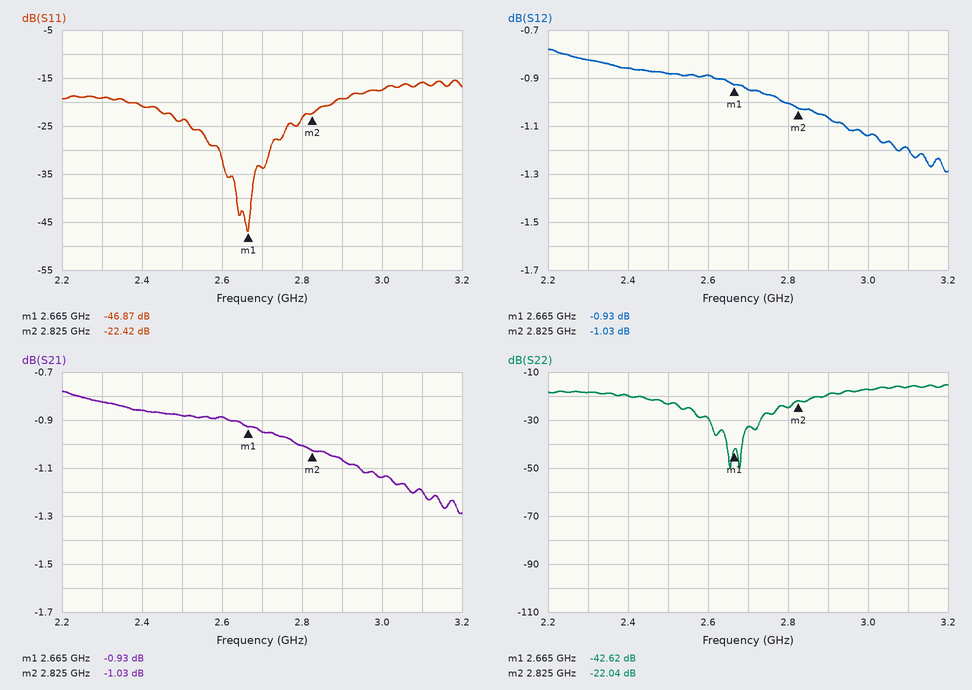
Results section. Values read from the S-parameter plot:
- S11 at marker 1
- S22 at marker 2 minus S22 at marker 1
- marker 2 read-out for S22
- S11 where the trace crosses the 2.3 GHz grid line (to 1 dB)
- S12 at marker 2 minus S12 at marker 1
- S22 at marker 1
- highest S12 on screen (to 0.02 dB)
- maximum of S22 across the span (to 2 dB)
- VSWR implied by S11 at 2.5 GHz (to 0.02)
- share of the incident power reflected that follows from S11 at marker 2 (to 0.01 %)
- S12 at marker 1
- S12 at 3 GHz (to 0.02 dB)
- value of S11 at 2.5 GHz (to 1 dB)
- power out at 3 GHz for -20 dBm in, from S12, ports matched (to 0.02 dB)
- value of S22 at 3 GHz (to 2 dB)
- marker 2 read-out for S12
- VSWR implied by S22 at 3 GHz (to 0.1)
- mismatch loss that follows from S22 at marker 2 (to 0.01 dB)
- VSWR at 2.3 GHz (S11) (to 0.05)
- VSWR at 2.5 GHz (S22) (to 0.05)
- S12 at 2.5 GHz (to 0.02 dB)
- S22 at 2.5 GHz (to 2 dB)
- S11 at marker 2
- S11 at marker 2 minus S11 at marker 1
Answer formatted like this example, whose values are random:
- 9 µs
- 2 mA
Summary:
- -46.87 dB
- 20.58 dB
- -22.04 dB
- -19 dB
- -0.10 dB
- -42.62 dB
- -0.78 dB
- -16 dB
- 1.14
- 0.57 %
- -0.93 dB
- -1.14 dB
- -24 dB
- -21.14 dBm
- -18 dB
- -1.03 dB
- 1.3
- 0.03 dB
- 1.25
- 1.15
- -0.88 dB
- -24 dB
- -22.42 dB
- 24.45 dB
